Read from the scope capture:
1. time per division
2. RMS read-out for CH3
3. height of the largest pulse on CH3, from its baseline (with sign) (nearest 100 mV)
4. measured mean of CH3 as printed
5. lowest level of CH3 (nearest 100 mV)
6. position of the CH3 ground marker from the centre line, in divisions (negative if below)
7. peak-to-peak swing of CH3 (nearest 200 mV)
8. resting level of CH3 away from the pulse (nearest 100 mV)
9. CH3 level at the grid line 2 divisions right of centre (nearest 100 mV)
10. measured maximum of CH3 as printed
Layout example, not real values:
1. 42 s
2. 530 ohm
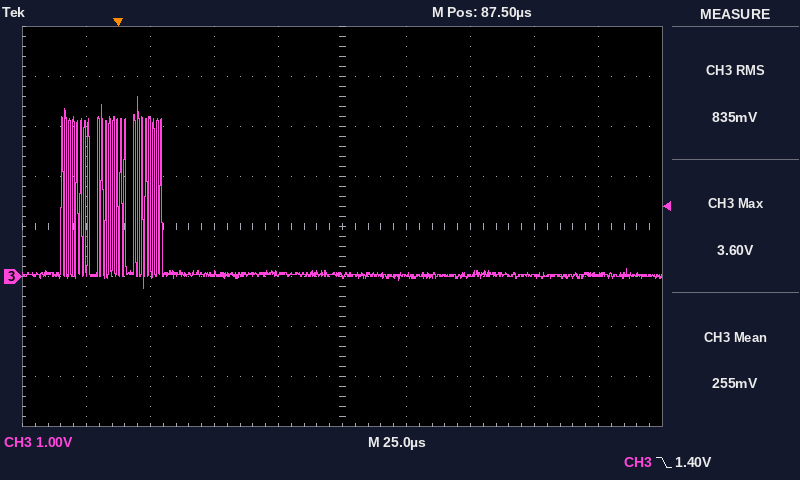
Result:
1. 25 µs
2. 835 mV
3. +3.6 V
4. 255 mV
5. -200 mV
6. -1.0 div
7. 3.8 V
8. 0.0 V
9. 0.0 V
10. 3.60 V
